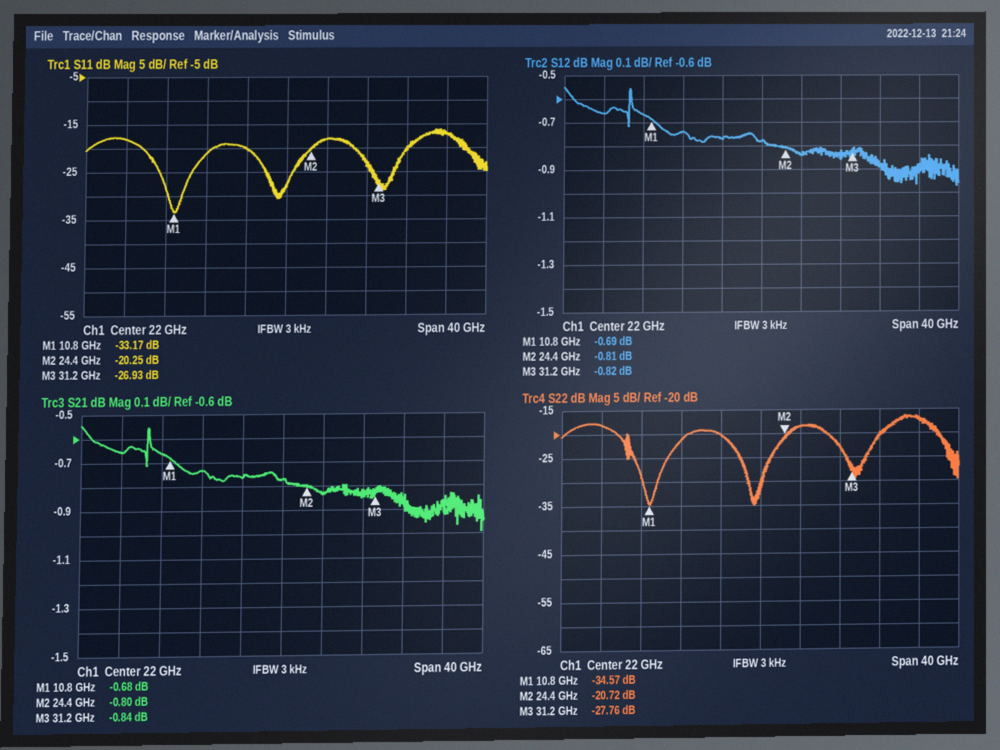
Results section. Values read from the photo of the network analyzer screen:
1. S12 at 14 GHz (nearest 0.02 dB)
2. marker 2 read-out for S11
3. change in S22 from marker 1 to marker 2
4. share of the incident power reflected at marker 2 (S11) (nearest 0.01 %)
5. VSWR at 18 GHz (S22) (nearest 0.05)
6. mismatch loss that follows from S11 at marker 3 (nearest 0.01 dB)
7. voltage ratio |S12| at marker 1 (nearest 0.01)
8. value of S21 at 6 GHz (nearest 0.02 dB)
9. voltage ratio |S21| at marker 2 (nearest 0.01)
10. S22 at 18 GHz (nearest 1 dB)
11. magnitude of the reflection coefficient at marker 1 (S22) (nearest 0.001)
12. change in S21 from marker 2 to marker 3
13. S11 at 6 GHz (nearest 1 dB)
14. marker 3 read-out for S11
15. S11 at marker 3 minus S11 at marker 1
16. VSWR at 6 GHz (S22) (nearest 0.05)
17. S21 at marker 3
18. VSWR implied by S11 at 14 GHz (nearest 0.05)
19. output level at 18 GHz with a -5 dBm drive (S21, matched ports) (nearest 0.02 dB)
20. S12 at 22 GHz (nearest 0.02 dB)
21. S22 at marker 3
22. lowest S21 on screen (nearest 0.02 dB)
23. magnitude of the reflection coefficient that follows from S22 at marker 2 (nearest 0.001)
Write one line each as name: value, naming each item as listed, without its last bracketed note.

S12 at 14 GHz: -0.74 dB
marker 2 read-out for S11: -20.25 dB
change in S22 from marker 1 to marker 2: 13.85 dB
share of the incident power reflected at marker 2 (S11): 0.94 %
VSWR at 18 GHz (S22): 1.20
mismatch loss that follows from S11 at marker 3: 0.01 dB
voltage ratio |S12| at marker 1: 0.92
value of S21 at 6 GHz: -0.66 dB
voltage ratio |S21| at marker 2: 0.91
S22 at 18 GHz: -20 dB
magnitude of the reflection coefficient at marker 1 (S22): 0.019
change in S21 from marker 2 to marker 3: -0.04 dB
S11 at 6 GHz: -18 dB
marker 3 read-out for S11: -26.93 dB
S11 at marker 3 minus S11 at marker 1: 6.24 dB
VSWR at 6 GHz (S22): 1.30
S21 at marker 3: -0.84 dB
VSWR implied by S11 at 14 GHz: 1.20
output level at 18 GHz with a -5 dBm drive (S21, matched ports): -5.76 dBm
S12 at 22 GHz: -0.78 dB
S22 at marker 3: -27.76 dB
lowest S21 on screen: -1.00 dB
magnitude of the reflection coefficient that follows from S22 at marker 2: 0.092
